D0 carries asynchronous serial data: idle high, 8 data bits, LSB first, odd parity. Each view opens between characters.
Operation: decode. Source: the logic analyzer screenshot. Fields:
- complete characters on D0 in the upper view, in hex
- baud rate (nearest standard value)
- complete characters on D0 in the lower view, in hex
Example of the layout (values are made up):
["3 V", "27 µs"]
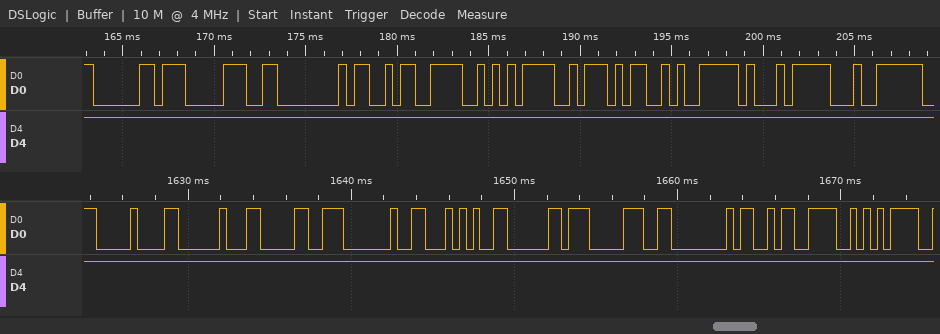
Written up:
["60, 70, 80, 9A, AA, BA, CA, D1, E4", "2400 baud", "10, 20, 30, 40, 54, 60, 70, 80, 9A, AA"]
